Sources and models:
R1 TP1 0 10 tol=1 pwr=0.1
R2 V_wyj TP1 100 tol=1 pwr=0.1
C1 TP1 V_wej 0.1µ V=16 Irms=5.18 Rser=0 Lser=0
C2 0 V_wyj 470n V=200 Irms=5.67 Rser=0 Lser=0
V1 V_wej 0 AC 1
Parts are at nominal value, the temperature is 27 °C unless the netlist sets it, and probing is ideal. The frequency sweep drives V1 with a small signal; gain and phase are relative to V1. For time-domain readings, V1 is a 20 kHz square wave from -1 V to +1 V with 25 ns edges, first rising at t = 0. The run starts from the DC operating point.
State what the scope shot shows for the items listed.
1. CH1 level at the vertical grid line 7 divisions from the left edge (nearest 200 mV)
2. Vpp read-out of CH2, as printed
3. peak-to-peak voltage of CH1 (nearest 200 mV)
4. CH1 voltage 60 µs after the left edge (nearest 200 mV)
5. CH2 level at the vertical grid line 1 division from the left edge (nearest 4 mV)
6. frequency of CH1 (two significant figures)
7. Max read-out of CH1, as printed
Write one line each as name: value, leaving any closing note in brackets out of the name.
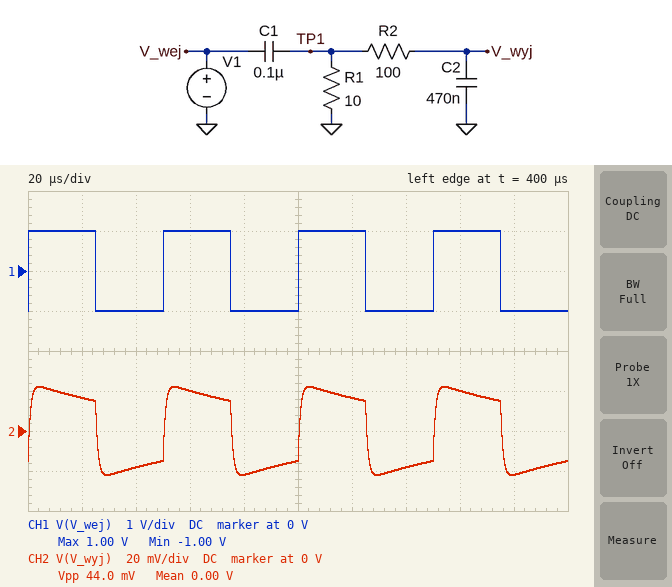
CH1 level at the vertical grid line 7 divisions from the left edge: -1.0 V
Vpp read-out of CH2, as printed: 44.0 mV
peak-to-peak voltage of CH1: 2.0 V
CH1 voltage 60 µs after the left edge: 1.0 V
CH2 level at the vertical grid line 1 division from the left edge: 16 mV
frequency of CH1: 20 kHz
Max read-out of CH1, as printed: 1.00 V
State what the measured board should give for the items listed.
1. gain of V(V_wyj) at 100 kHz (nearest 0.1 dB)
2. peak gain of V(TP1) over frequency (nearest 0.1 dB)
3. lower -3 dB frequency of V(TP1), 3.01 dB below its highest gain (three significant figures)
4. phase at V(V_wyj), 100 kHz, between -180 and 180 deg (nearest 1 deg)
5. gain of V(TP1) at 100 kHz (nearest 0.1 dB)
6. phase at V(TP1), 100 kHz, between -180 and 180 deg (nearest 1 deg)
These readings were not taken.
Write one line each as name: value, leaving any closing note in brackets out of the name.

gain of V(V_wyj) at 100 kHz: -35.5 dB
peak gain of V(TP1) over frequency: 0 dB
lower -3 dB frequency of V(TP1), 3.01 dB below its highest gain: 175 kHz
phase at V(V_wyj), 100 kHz, between -180 and 180 deg: -28 deg
gain of V(TP1) at 100 kHz: -6.1 dB
phase at V(TP1), 100 kHz, between -180 and 180 deg: 60 deg
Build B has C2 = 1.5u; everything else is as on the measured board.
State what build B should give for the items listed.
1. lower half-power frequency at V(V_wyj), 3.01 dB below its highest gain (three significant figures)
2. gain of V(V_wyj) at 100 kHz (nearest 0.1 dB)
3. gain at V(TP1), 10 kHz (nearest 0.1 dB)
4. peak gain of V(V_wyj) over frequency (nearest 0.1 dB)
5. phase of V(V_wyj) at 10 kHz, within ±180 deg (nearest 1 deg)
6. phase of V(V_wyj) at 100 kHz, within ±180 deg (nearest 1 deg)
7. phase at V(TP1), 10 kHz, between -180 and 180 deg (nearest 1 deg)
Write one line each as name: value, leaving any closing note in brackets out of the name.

lower half-power frequency at V(V_wyj), 3.01 dB below its highest gain: 954 Hz
gain of V(V_wyj) at 100 kHz: -45.6 dB
gain at V(TP1), 10 kHz: -24.9 dB
peak gain of V(V_wyj) over frequency: -44.4 dB
phase of V(V_wyj) at 10 kHz, within ±180 deg: 2 deg
phase of V(V_wyj) at 100 kHz, within ±180 deg: -29 deg
phase at V(TP1), 10 kHz, between -180 and 180 deg: 86 deg
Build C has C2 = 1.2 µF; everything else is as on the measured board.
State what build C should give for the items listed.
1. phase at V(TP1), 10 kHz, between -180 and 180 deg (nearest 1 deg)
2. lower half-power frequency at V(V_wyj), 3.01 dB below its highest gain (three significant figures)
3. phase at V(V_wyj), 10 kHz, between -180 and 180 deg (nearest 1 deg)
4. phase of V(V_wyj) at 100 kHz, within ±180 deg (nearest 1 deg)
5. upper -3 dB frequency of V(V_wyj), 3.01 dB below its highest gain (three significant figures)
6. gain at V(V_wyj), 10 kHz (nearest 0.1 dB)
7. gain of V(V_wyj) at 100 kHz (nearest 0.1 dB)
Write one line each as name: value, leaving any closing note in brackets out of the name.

phase at V(TP1), 10 kHz, between -180 and 180 deg: 86 deg
lower half-power frequency at V(V_wyj), 3.01 dB below its highest gain: 1.19 kHz
phase at V(V_wyj), 10 kHz, between -180 and 180 deg: 4 deg
phase of V(V_wyj) at 100 kHz, within ±180 deg: -29 deg
upper -3 dB frequency of V(V_wyj), 3.01 dB below its highest gain: 178 kHz
gain at V(V_wyj), 10 kHz: -42.5 dB
gain of V(V_wyj) at 100 kHz: -43.6 dB
